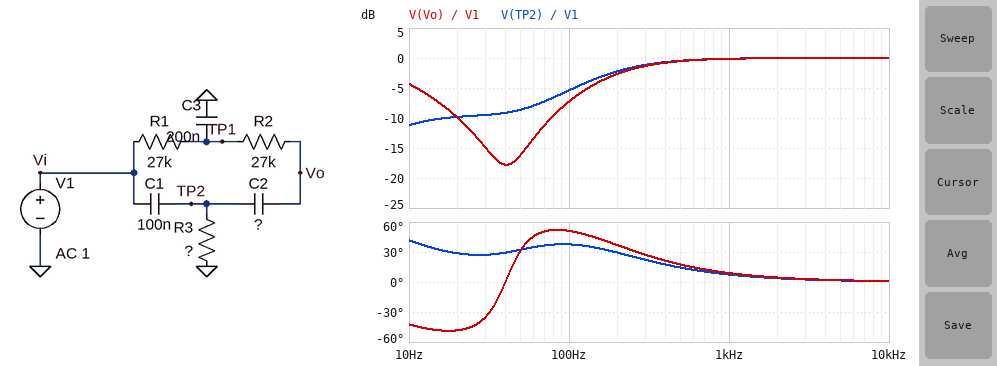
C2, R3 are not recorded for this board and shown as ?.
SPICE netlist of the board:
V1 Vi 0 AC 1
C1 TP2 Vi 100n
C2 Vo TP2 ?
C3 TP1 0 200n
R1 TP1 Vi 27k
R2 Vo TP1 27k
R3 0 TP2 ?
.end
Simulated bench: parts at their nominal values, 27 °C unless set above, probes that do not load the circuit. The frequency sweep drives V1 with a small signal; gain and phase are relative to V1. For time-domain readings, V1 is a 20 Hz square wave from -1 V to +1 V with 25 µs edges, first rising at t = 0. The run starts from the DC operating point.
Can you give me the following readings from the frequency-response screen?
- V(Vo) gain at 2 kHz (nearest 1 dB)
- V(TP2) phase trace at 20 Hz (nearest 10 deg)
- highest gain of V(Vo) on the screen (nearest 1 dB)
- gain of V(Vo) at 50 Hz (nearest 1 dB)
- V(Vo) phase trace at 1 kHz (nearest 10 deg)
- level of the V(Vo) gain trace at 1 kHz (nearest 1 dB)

0 dB
30 deg
0 dB
-16 dB
10 deg
0 dB
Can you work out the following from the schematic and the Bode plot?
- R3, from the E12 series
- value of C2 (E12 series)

22 kΩ
220 nF
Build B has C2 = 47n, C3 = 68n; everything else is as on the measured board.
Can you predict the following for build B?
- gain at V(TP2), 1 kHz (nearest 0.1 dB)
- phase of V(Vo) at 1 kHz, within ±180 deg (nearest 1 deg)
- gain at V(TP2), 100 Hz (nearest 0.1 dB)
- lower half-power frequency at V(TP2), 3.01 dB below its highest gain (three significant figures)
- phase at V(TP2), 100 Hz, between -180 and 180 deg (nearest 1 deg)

-0.2 dB
14 deg
-3.3 dB
119 Hz
27 deg
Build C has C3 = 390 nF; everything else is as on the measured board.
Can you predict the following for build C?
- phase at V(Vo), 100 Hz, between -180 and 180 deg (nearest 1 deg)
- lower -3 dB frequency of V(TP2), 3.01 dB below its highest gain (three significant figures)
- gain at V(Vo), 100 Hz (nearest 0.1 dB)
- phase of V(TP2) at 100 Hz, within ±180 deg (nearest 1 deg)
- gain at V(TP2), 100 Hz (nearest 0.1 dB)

59 deg
155 Hz
-6.4 dB
43 deg
-5.3 dB
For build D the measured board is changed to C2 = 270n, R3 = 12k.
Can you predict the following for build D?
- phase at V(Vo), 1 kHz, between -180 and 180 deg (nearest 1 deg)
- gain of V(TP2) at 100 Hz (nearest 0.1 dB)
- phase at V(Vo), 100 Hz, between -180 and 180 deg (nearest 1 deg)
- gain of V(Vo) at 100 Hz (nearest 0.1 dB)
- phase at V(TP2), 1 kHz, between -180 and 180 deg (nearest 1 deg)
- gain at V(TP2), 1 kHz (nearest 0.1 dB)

12 deg
-7.6 dB
63 deg
-9.3 dB
11 deg
-0.2 dB
